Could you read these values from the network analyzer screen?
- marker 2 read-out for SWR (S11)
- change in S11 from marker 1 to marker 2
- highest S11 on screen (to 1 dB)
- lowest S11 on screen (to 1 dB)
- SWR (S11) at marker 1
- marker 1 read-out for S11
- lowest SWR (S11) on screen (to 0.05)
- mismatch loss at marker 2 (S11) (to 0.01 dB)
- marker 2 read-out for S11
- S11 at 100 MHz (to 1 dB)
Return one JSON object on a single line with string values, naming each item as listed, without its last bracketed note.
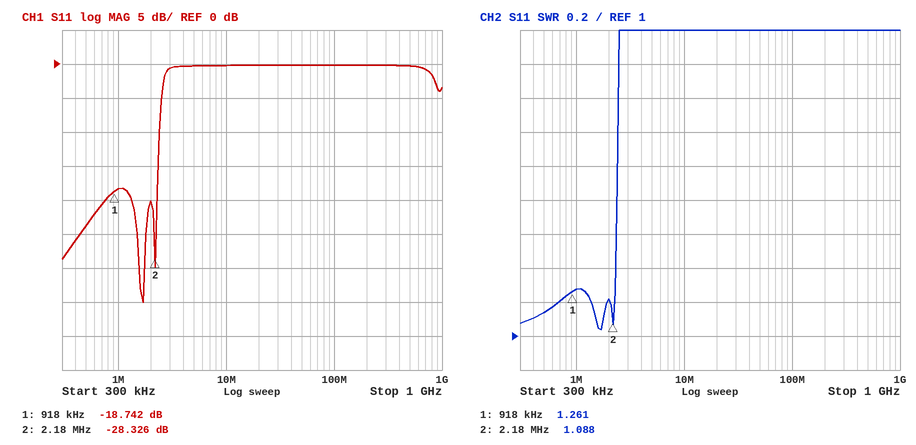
{"marker 2 read-out for SWR": "1.088", "change in S11 from marker 1 to marker 2": "-9.584 dB", "highest S11 on screen": "0 dB", "lowest S11 on screen": "-35 dB", "SWR (S11) at marker 1": "1.261", "marker 1 read-out for S11": "-18.742 dB", "lowest SWR (S11) on screen": "1.05", "mismatch loss at marker 2 (S11)": "0.01 dB", "marker 2 read-out for S11": "-28.326 dB", "S11 at 100 MHz": "0 dB"}
